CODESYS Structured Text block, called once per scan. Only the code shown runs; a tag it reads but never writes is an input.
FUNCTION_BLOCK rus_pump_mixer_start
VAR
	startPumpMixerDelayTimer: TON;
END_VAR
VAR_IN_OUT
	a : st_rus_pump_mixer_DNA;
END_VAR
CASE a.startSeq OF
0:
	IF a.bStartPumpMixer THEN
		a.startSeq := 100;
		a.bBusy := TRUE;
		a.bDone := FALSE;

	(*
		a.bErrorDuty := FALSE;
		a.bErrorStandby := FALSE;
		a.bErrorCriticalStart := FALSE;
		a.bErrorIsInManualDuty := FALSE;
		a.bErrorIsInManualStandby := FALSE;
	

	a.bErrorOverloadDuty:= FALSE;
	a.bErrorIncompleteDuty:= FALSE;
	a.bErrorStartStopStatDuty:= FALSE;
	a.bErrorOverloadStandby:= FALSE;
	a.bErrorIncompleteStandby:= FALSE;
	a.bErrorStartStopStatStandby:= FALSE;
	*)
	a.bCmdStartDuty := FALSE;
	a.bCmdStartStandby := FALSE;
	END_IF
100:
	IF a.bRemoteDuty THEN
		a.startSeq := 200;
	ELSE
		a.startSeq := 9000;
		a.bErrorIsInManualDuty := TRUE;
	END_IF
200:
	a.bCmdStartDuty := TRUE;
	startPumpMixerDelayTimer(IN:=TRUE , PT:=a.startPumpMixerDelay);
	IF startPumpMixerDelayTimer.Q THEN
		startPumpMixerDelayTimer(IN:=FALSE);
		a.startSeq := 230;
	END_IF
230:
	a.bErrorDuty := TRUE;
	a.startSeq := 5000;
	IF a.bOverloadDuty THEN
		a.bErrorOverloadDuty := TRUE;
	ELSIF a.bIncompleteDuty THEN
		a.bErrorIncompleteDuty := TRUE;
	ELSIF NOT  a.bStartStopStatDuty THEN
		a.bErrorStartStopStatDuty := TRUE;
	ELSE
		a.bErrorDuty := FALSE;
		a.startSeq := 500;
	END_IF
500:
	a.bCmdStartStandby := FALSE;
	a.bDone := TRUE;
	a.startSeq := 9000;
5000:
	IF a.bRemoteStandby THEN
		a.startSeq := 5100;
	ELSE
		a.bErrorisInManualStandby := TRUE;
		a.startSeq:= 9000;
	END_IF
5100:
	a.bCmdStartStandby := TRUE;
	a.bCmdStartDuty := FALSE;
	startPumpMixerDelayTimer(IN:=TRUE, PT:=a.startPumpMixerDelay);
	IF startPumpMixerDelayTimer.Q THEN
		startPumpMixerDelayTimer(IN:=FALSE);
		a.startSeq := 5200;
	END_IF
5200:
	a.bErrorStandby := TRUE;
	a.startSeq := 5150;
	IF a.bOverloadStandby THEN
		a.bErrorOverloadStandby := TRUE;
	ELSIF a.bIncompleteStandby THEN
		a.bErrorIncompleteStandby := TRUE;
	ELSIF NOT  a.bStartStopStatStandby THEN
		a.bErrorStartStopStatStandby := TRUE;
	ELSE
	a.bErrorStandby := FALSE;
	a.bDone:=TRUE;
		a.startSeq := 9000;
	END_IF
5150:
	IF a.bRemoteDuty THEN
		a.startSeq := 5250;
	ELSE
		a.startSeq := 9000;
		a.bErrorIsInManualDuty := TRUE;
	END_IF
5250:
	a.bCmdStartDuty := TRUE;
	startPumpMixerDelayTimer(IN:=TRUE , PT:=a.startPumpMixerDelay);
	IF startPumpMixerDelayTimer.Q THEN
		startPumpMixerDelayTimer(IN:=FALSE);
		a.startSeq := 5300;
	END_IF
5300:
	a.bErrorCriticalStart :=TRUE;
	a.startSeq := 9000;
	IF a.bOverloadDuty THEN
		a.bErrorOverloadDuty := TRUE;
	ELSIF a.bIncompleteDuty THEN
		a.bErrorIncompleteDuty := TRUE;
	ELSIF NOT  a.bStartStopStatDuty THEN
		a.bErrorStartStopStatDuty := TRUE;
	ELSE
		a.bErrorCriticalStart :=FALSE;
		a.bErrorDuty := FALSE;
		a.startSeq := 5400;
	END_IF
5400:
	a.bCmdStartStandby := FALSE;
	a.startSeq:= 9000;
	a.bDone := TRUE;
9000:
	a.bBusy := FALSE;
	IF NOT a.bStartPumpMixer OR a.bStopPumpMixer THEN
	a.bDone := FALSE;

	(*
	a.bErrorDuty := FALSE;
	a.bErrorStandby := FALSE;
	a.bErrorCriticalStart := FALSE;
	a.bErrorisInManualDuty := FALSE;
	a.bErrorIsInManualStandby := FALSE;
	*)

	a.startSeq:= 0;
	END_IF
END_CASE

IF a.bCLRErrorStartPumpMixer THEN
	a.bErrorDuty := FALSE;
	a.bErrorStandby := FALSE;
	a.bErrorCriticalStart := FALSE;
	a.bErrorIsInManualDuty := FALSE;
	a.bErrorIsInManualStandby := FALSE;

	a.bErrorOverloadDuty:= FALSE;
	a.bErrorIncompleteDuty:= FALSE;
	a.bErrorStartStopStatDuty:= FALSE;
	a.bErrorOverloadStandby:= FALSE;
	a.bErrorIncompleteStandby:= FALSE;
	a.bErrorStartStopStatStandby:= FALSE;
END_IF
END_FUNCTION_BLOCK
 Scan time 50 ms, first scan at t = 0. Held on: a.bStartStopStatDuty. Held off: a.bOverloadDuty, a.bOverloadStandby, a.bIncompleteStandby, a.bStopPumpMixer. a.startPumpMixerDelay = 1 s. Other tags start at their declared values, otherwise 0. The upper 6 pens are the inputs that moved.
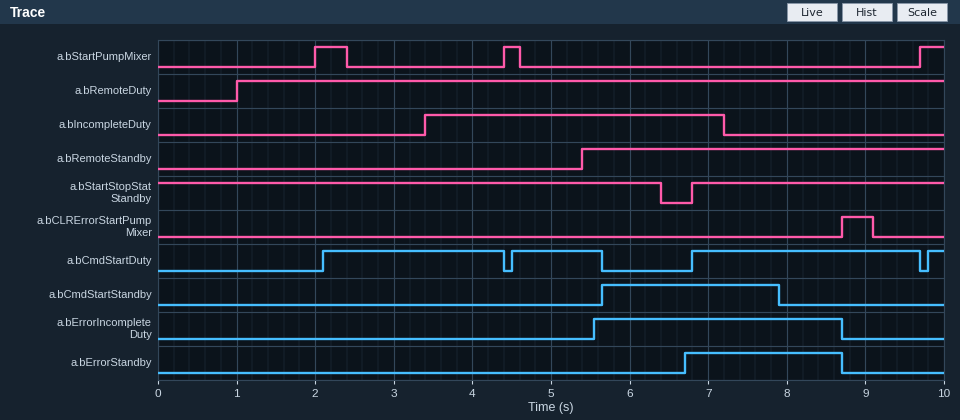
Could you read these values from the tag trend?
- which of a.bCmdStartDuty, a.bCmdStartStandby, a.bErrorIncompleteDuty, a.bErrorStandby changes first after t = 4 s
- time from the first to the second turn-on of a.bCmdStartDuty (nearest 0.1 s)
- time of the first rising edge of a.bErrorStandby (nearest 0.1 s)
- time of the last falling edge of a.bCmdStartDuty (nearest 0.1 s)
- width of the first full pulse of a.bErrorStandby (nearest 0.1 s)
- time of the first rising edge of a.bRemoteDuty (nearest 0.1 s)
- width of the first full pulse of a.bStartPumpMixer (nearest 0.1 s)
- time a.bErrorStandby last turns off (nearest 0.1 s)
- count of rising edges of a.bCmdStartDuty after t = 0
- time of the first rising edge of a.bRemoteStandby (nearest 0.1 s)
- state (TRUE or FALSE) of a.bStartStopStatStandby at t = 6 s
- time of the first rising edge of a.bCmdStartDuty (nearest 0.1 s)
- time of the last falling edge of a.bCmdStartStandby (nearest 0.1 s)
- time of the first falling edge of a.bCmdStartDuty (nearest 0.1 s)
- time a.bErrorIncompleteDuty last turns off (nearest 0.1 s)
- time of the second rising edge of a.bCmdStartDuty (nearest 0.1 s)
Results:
a.bCmdStartDuty
2.4 s
6.7 s
9.7 s
2.0 s
1.0 s
0.4 s
8.7 s
4
5.4 s
TRUE
2.1 s
7.9 s
4.4 s
8.7 s
4.5 s
